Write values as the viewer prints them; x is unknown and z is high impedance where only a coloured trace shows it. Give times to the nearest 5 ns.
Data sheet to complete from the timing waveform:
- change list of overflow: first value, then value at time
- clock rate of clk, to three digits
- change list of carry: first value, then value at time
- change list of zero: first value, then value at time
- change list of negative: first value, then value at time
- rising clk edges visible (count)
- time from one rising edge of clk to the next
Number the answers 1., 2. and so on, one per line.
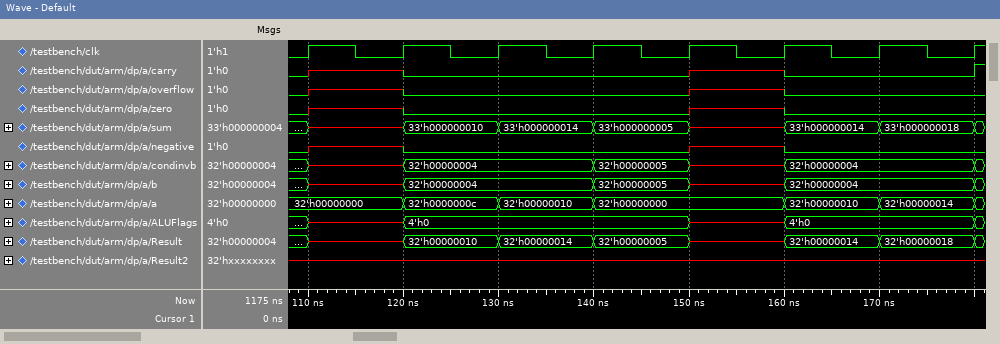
1. 0, x at 110 ns, 0 at 120 ns, x at 150 ns, 0 at 160 ns
2. 100 MHz
3. 0, x at 110 ns, 0 at 120 ns, x at 150 ns, 0 at 160 ns, 1 at 180 ns
4. 0, x at 110 ns, 0 at 120 ns, x at 150 ns, 0 at 160 ns
5. 0, x at 110 ns, 0 at 120 ns, x at 150 ns, 0 at 160 ns
6. 8
7. 10 ns
